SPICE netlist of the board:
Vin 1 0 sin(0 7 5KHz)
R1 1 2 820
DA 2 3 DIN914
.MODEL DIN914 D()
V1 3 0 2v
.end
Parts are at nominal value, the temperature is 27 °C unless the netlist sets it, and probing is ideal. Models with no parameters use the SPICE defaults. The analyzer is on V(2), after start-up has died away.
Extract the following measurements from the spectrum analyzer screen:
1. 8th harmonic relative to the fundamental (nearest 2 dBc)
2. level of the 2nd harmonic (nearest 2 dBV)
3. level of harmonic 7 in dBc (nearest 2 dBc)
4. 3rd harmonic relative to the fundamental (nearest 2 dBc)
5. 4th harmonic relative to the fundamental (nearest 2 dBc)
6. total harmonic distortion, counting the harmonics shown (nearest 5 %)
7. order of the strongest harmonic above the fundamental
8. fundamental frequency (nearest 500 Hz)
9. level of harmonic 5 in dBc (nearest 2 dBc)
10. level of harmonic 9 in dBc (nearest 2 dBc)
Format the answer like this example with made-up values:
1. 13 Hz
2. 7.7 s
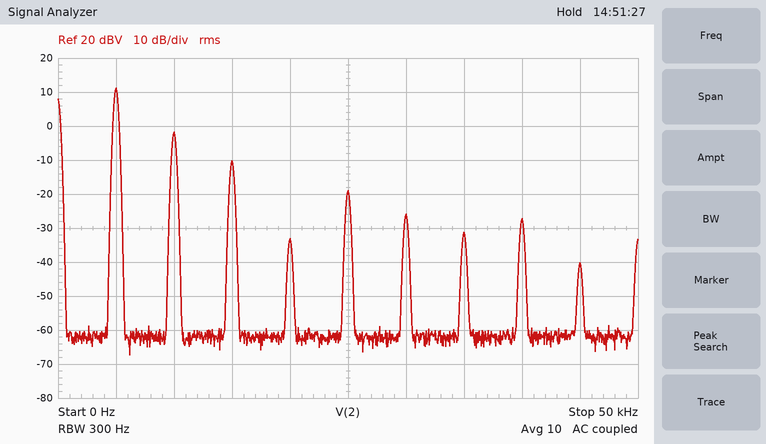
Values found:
1. -38 dBc
2. -2 dBV
3. -42 dBc
4. -22 dBc
5. -44 dBc
6. 25 %
7. 2
8. 5.0 kHz
9. -30 dBc
10. -52 dBc
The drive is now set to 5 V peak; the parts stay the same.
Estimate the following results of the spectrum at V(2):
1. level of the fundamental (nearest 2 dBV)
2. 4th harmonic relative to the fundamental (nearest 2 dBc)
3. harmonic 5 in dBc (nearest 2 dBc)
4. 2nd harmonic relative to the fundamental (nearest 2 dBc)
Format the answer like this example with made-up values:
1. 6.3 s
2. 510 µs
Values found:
1. 10 dBV
2. -34 dBc
3. -38 dBc
4. -16 dBc
